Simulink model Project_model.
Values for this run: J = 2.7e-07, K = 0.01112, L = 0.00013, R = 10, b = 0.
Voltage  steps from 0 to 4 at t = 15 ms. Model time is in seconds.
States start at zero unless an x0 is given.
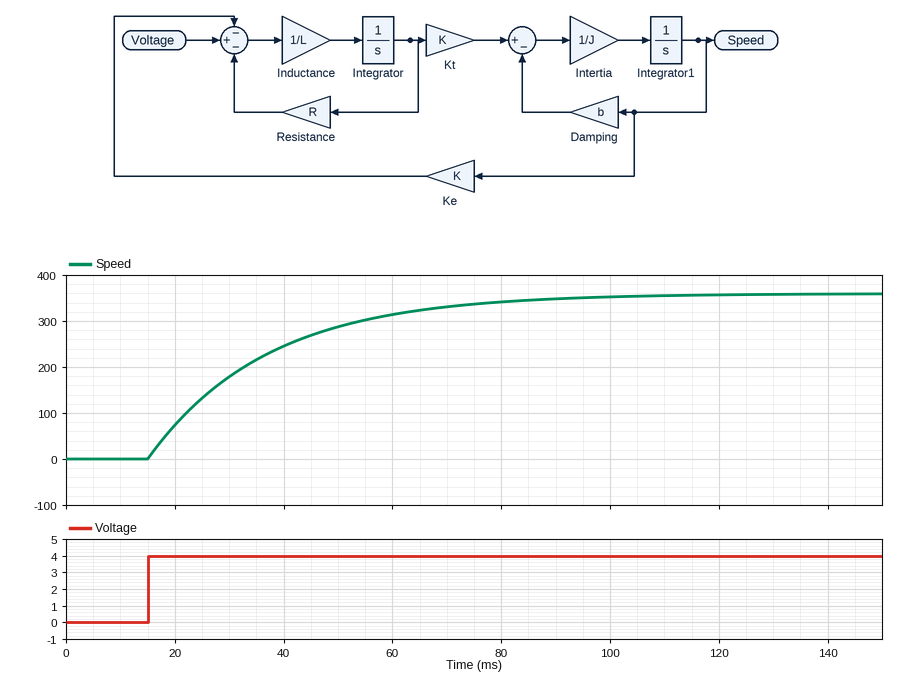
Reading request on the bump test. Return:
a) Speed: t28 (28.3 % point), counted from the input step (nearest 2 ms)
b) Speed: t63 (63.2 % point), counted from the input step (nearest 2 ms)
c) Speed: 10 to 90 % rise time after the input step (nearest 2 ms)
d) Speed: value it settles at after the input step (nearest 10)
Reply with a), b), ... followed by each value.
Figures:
a) 8 ms
b) 22 ms
c) 48 ms
d) 360
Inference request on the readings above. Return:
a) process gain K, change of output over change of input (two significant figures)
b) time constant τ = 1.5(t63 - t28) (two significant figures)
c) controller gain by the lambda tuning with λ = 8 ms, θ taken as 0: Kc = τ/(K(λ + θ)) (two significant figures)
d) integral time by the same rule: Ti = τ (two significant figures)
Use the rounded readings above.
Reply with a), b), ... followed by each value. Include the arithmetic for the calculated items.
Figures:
a) (360 - 0) / 4 = 90
b) 1.5 × (22 - 8) = 21 ms
c) 21 / (90 × (8 + 0)) = 0.029
d) 21 ms
